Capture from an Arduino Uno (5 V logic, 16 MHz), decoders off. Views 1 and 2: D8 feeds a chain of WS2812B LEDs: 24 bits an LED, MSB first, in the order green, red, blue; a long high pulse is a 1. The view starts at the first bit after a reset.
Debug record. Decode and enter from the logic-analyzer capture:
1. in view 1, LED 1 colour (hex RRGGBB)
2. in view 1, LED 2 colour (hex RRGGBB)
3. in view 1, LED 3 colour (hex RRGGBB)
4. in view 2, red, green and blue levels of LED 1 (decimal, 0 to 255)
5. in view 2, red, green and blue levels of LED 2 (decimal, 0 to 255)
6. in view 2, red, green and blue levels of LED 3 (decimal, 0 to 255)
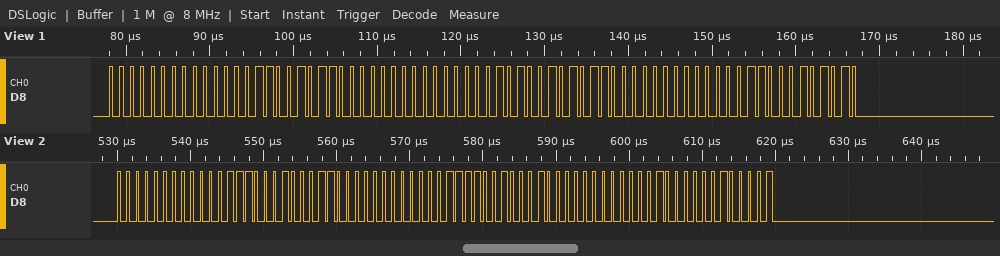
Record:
#03002C
#05002B
#06002A
14, 0, 35
15, 0, 34
16, 0, 33
